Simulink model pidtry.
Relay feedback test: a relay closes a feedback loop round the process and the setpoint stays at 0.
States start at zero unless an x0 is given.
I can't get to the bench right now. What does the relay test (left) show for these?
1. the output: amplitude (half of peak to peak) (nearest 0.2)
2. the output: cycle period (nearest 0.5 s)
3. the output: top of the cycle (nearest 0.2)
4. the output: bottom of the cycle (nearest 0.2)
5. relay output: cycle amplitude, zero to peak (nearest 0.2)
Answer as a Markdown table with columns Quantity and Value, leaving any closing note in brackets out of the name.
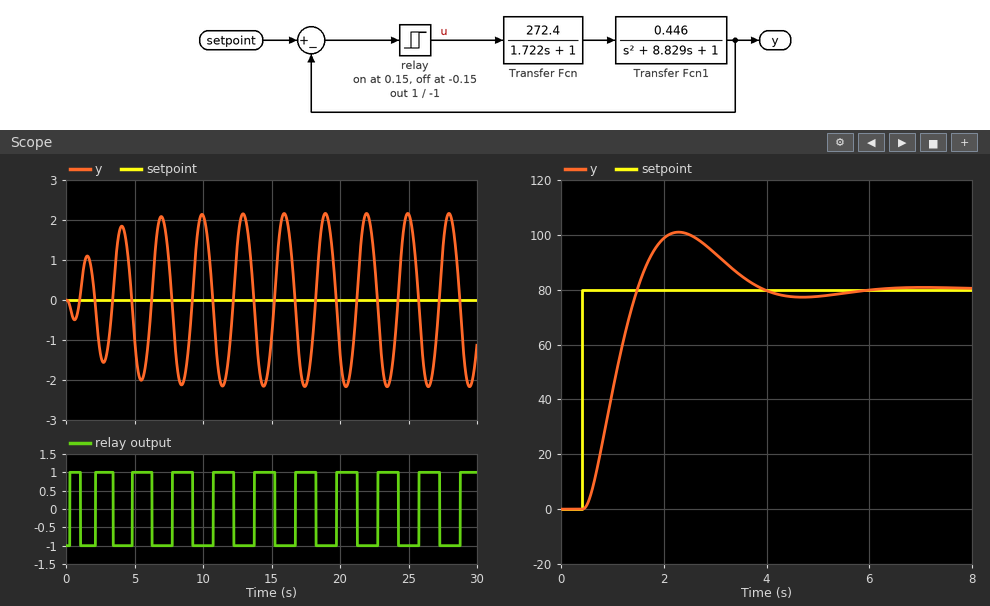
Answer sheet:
| Quantity | Value |
|---|---|
| the output: amplitude (half of peak to peak) | 2.2 |
| the output: cycle period | 3.0 s |
| the output: top of the cycle | 2.2 |
| the output: bottom of the cycle | -2.2 |
| relay output: cycle amplitude, zero to peak | 1.0 |
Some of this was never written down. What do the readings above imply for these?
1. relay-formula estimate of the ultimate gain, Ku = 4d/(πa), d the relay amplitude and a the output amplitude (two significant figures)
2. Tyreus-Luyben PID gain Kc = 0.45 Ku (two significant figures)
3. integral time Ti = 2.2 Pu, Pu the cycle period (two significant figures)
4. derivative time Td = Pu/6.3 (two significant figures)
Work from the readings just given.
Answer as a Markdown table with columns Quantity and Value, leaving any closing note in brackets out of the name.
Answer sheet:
| Quantity | Value |
|---|---|
| relay-formula estimate of the ultimate gain, Ku = 4d/(πa), d the relay amplitude and a the output amplitude | 0.58 |
| Tyreus-Luyben PID gain Kc = 0.45 Ku | 0.26 |
| integral time Ti = 2.2 Pu, Pu the cycle period | 6.6 s |
| derivative time Td = Pu/6.3 | 0.48 s |
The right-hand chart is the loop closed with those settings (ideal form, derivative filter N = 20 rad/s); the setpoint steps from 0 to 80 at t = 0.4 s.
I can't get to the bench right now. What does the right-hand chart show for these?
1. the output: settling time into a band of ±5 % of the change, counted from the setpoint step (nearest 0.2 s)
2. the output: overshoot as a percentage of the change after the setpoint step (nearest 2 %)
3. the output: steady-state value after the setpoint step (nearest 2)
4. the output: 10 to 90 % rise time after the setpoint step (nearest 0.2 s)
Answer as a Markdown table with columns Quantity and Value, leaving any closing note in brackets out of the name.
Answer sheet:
| Quantity | Value |
|---|---|
| the output: settling time into a band of ±5 % of the change, counted from the setpoint step | 3.2 s |
| the output: overshoot as a percentage of the change after the setpoint step | 26 % |
| the output: steady-state value after the setpoint step | 80 |
| the output: 10 to 90 % rise time after the setpoint step | 0.8 s |
